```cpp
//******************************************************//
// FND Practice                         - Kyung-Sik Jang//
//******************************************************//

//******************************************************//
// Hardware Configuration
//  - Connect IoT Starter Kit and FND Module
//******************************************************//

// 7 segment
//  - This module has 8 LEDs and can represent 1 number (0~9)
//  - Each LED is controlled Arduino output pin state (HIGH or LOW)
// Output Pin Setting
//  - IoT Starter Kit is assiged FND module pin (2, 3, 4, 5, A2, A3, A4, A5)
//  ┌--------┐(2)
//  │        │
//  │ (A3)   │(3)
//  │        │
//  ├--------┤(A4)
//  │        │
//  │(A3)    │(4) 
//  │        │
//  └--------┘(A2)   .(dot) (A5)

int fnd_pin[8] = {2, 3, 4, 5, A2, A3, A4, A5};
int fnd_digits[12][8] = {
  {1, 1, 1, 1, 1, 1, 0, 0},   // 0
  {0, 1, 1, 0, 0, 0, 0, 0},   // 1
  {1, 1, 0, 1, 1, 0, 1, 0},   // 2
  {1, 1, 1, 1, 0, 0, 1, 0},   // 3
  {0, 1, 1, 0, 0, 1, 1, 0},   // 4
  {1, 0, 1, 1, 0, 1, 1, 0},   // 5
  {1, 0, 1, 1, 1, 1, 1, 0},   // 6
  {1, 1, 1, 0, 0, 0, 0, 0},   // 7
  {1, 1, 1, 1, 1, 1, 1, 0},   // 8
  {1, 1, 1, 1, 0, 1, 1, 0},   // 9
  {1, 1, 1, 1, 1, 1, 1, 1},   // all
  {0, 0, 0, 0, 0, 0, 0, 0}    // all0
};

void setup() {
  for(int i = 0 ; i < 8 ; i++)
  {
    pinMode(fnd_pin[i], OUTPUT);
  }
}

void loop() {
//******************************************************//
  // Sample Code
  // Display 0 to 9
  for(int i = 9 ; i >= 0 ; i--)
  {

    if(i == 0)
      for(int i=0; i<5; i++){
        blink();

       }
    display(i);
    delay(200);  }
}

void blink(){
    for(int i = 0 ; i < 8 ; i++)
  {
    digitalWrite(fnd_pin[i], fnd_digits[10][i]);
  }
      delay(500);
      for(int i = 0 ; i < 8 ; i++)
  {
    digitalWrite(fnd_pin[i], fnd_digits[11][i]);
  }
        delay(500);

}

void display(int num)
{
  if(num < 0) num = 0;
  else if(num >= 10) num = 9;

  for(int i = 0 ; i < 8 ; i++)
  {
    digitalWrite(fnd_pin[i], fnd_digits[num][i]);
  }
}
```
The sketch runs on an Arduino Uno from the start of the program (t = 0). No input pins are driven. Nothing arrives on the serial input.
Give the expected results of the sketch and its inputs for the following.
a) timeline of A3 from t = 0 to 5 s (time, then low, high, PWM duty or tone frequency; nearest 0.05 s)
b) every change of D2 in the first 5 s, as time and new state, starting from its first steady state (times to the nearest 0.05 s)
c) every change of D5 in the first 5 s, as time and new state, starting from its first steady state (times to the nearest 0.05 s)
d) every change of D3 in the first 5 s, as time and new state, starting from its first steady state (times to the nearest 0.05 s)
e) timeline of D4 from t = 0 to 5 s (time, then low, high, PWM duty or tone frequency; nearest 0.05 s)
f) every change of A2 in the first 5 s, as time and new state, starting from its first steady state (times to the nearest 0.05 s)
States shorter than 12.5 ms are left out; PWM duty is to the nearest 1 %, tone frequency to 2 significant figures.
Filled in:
0 s high; 0.4 s low; 0.6 s high; 1.2 s low; 1.8 s high; 2.3 s low; 2.8 s high; 3.3 s low; 3.8 s high; 4.3 s low; 4.8 s high
0 s high; 1 s low; 1.2 s high; 1.6 s low; 1.8 s high; 2.3 s low; 2.8 s high; 3.3 s low; 3.8 s high; 4.3 s low; 4.8 s high
0 s high; 0.4 s low; 0.6 s high; 1 s low; 1.2 s high; 1.6 s low; 1.8 s high; 2.3 s low; 2.8 s high; 3.3 s low; 3.8 s high; 4.3 s low; 4.8 s high
0 s high; 0.6 s low; 1 s high; 2.3 s low; 2.8 s high; 3.3 s low; 3.8 s high; 4.3 s low; 4.8 s high
0 s high; 1.4 s low; 1.6 s high; 2.3 s low; 2.8 s high; 3.3 s low; 3.8 s high; 4.3 s low; 4.8 s high
0 s low; 0.2 s high; 0.4 s low; 0.6 s high; 0.8 s low; 1.4 s high; 1.6 s low; 1.8 s high; 2.3 s low; 2.8 s high; 3.3 s low; 3.8 s high; 4.3 s low; 4.8 s high
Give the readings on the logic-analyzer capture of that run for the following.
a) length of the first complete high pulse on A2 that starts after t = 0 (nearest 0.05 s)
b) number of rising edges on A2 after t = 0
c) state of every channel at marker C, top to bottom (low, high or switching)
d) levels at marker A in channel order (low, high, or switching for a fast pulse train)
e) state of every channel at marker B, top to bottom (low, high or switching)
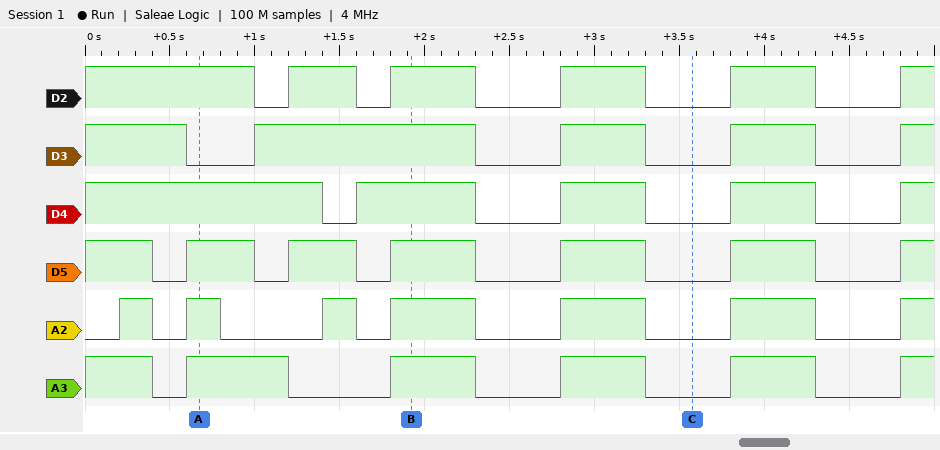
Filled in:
0.20 s
7
D2 low, D3 low, D4 low, D5 low, A2 low, A3 low
D2 high, D3 low, D4 high, D5 high, A2 high, A3 high
D2 high, D3 high, D4 high, D5 high, A2 high, A3 high
